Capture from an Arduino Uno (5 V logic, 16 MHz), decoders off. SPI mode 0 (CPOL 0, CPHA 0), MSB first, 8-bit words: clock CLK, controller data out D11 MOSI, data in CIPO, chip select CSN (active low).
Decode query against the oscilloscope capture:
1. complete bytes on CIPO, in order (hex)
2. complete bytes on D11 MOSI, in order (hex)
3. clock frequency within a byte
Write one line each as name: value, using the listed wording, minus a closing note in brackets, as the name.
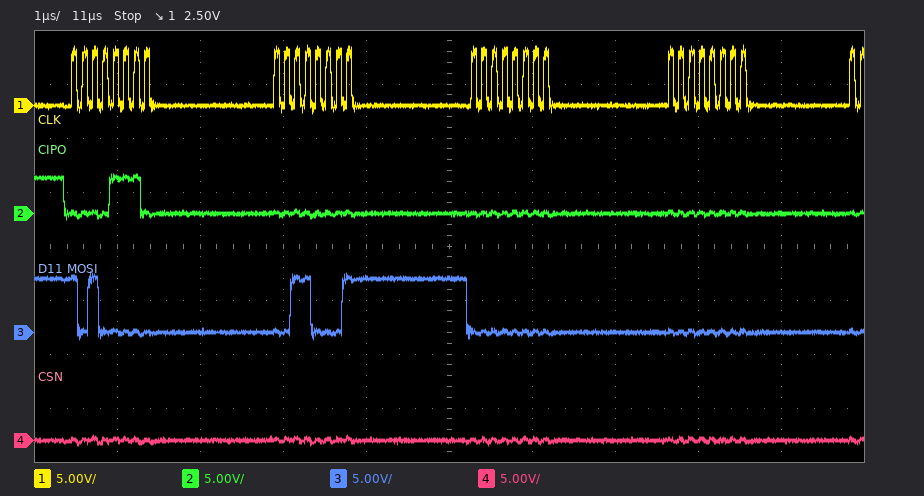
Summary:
complete bytes on CIPO, in order: 0E 00 00 00
complete bytes on D11 MOSI, in order: A0 31 00 00
clock frequency within a byte: 8 MHz
